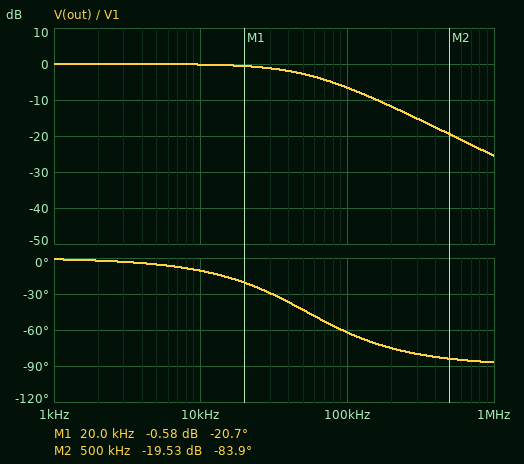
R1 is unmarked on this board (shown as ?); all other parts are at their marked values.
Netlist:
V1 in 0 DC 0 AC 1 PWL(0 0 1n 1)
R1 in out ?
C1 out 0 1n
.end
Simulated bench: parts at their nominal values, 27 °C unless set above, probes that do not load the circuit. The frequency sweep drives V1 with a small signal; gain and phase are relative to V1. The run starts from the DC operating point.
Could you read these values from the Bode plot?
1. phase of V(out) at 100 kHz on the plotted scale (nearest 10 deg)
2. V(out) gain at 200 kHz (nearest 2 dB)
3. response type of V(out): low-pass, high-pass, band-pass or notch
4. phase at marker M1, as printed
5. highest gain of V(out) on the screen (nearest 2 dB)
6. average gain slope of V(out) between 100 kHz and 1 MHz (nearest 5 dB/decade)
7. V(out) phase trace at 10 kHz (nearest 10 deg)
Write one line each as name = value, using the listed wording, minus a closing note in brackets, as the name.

phase of V(out) at 100 kHz on the plotted scale = -60 deg
V(out) gain at 200 kHz = -12 dB
response type of V(out): low-pass, high-pass, band-pass or notch = low-pass
phase at marker M1, as printed = -20.7 deg
highest gain of V(out) on the screen = 0 dB
average gain slope of V(out) between 100 kHz and 1 MHz = -20 dB/decade
V(out) phase trace at 10 kHz = -10 deg
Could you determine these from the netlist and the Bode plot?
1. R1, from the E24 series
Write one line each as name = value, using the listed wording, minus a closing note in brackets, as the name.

R1, from the E24 series = 3 kΩ
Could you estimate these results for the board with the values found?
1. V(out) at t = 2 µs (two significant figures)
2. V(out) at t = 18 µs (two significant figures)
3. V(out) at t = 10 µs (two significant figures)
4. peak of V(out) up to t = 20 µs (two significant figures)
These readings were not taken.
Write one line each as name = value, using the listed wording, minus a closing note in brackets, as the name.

V(out) at t = 2 µs = 490 mV
V(out) at t = 18 µs = 1.0 V
V(out) at t = 10 µs = 960 mV
peak of V(out) up to t = 20 µs = 1.0 V
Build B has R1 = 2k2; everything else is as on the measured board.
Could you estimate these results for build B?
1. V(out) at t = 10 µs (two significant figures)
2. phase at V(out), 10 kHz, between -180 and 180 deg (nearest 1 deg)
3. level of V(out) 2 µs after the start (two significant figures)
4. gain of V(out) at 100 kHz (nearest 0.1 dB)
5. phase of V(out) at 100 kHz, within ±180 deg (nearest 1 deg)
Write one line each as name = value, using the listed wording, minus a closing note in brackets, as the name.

V(out) at t = 10 µs = 990 mV
phase at V(out), 10 kHz, between -180 and 180 deg = -8 deg
level of V(out) 2 µs after the start = 600 mV
gain of V(out) at 100 kHz = -4.6 dB
phase of V(out) at 100 kHz, within ±180 deg = -54 deg
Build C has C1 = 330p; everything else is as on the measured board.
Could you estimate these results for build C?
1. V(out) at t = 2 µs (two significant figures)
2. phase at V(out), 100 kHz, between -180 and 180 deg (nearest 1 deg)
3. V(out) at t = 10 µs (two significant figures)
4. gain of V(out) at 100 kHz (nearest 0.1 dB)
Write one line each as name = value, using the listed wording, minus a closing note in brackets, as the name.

V(out) at t = 2 µs = 870 mV
phase at V(out), 100 kHz, between -180 and 180 deg = -32 deg
V(out) at t = 10 µs = 1.0 V
gain of V(out) at 100 kHz = -1.4 dB
